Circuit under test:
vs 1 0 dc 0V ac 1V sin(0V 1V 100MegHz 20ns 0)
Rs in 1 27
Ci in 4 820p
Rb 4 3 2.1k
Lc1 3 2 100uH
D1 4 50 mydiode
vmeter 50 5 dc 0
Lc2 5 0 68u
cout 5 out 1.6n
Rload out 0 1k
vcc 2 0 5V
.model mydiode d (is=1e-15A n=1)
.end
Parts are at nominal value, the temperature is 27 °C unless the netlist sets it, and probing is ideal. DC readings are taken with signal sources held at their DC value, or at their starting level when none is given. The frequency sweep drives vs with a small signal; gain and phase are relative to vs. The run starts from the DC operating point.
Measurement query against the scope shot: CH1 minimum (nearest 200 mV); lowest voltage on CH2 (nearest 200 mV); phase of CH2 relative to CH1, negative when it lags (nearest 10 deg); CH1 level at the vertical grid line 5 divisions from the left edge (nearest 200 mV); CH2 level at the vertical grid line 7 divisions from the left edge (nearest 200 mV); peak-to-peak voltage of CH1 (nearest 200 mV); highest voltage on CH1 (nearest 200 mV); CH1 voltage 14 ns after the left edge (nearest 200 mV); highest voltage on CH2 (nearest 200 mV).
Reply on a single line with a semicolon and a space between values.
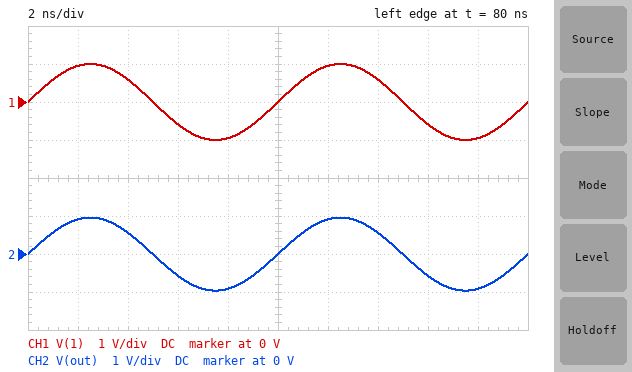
-1.0 V; -1.0 V; 0 deg; 0 V; 600 mV; 2.0 V; 1.0 V; 600 mV; 1.0 V
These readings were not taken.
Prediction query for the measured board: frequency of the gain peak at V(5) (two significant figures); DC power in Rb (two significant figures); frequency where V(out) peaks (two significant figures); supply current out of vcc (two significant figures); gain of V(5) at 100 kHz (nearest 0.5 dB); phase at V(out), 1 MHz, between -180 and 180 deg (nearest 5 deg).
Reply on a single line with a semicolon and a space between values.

710 kHz; 8.7 mW; 710 kHz; 2.0 mA; -33.0 dB; 40 deg
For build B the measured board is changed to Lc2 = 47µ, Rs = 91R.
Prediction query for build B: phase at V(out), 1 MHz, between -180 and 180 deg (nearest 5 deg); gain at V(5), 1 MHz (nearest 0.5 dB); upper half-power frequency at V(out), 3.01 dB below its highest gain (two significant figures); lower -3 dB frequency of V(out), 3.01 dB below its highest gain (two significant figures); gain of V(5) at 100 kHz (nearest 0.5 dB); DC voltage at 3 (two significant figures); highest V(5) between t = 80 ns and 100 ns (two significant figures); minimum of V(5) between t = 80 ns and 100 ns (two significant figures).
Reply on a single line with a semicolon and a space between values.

60 deg; 2.0 dB; 7.3 MHz; 640 kHz; -36.0 dB; 5.0 V; 900 mV; -910 mV
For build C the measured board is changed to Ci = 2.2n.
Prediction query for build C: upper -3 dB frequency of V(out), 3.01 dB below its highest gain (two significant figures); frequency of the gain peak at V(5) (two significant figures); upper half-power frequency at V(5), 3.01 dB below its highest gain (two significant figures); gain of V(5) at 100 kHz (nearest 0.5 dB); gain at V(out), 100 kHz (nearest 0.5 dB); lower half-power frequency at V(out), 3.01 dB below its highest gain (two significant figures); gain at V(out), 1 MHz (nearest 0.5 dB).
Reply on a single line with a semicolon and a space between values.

610 kHz; 420 kHz; 600 kHz; -24.0 dB; -27.0 dB; 340 kHz; 1.0 dB
